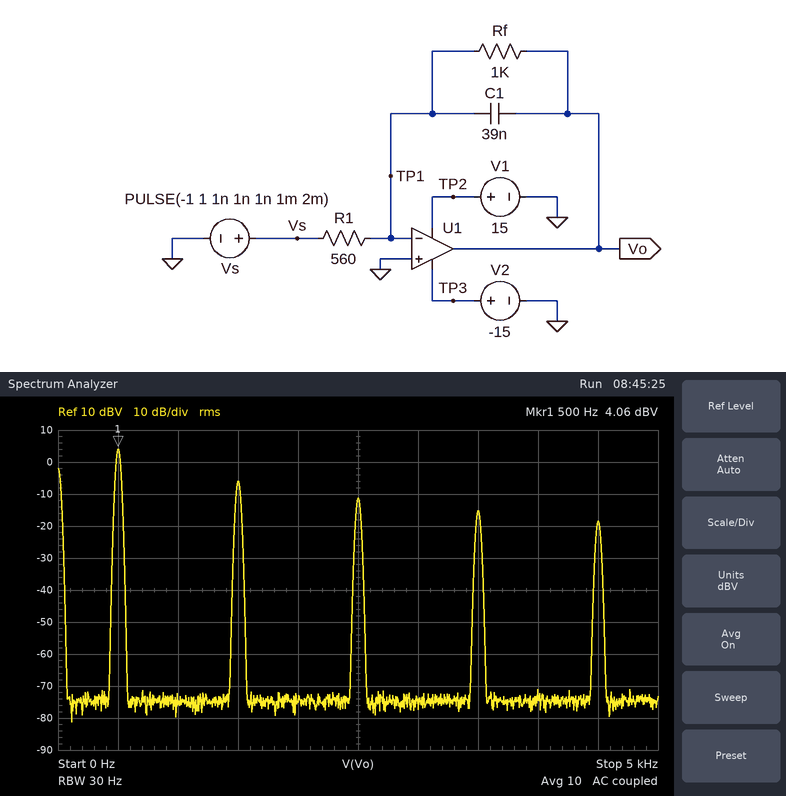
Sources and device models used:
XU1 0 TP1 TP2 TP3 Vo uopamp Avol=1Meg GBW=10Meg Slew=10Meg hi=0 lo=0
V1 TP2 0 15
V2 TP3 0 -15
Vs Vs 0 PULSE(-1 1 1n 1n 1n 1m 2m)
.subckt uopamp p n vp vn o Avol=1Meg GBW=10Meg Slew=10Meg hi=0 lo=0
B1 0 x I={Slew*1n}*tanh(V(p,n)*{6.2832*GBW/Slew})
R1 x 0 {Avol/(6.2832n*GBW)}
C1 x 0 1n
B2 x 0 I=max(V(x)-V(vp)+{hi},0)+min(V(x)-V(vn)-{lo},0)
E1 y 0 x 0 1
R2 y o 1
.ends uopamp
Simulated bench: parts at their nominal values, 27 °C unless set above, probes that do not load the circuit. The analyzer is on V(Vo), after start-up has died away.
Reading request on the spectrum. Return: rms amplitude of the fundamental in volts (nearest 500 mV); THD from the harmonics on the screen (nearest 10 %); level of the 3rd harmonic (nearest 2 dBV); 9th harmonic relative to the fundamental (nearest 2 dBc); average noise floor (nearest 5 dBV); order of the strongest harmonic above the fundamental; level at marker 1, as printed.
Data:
1.5 V
40 %
-6 dBV
-22 dBc
-75 dBV
3
4.06 dBV
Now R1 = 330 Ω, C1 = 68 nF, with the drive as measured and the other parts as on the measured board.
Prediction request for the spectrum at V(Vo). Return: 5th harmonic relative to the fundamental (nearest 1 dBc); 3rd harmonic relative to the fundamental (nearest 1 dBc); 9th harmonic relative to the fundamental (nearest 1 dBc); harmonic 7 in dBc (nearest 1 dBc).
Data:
-17 dBc
-11 dBc
-26 dBc
-22 dBc
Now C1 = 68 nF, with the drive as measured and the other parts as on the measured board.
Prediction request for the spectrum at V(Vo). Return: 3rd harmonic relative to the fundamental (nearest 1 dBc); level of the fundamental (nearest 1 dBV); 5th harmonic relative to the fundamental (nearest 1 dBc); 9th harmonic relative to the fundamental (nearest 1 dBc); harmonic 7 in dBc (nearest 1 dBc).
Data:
-11 dBc
4 dBV
-17 dBc
-26 dBc
-22 dBc
